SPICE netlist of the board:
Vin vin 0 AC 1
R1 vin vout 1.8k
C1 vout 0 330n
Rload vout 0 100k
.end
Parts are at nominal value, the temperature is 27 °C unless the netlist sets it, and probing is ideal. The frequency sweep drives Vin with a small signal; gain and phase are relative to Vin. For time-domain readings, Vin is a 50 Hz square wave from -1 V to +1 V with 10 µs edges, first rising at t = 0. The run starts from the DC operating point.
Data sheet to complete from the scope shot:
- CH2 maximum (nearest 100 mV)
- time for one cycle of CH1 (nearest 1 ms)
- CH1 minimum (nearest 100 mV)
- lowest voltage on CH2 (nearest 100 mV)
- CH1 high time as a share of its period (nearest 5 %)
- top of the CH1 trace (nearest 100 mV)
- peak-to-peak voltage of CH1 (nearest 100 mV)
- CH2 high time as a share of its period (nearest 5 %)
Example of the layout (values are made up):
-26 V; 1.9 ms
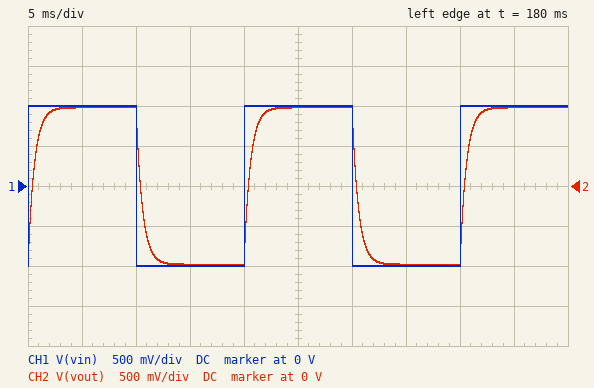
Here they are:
1.0 V; 20 ms; -1.0 V; -1.0 V; 50 %; 1.0 V; 2.0 V; 50 %
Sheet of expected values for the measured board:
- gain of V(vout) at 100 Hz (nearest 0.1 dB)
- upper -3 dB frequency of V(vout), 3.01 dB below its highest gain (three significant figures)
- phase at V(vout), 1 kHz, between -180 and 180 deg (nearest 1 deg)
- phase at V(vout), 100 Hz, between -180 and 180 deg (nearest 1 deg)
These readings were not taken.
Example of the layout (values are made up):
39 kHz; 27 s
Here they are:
-0.7 dB; 273 Hz; -75 deg; -20 deg
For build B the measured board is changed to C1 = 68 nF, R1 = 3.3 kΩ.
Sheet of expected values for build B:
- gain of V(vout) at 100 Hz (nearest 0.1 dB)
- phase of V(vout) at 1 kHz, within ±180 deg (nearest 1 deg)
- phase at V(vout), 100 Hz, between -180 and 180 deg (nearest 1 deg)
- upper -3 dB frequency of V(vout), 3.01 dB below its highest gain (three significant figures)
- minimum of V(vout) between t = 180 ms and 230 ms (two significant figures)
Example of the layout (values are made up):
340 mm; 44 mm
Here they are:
-0.4 dB; -54 deg; -8 deg; 733 Hz; -970 mV
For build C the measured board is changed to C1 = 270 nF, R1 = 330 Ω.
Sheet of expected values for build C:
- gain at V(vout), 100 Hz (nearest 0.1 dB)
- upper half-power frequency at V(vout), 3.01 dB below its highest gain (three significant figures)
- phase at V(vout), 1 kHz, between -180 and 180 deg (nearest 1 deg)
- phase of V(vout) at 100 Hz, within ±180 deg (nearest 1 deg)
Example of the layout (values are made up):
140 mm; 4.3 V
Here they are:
0 dB; 1.79 kHz; -29 deg; -3 deg
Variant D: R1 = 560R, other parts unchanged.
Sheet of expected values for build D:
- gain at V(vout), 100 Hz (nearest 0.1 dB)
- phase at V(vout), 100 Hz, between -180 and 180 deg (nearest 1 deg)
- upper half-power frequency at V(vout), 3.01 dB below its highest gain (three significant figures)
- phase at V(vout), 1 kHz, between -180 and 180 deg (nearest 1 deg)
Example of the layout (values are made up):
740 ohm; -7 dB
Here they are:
-0.1 dB; -7 deg; 866 Hz; -49 deg
